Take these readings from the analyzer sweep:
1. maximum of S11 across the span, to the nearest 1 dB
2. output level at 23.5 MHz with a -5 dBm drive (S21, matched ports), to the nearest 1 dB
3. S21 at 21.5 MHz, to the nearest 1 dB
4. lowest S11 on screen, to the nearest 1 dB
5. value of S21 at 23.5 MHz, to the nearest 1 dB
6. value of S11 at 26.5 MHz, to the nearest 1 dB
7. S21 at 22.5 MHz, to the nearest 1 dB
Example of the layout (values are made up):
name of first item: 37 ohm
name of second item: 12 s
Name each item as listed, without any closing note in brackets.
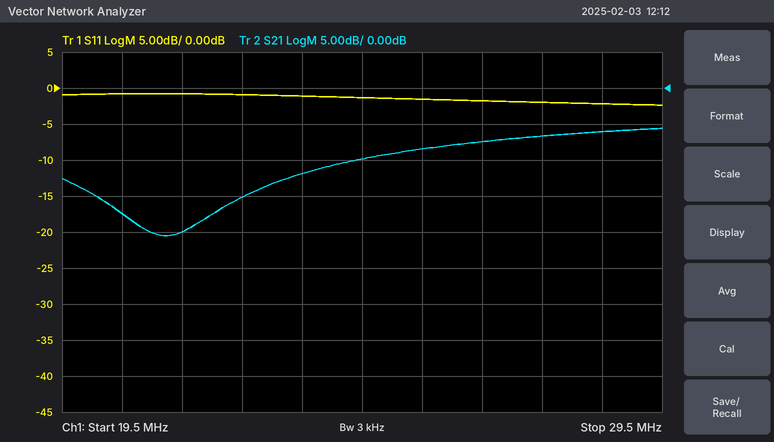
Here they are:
maximum of S11 across the span, to the nearest 1 dB: -1 dB
output level at 23.5 MHz with a -5 dBm drive (S21, matched ports), to the nearest 1 dB: -17 dBm
S21 at 21.5 MHz, to the nearest 1 dB: -20 dB
lowest S11 on screen, to the nearest 1 dB: -2 dB
value of S21 at 23.5 MHz, to the nearest 1 dB: -12 dB
value of S11 at 26.5 MHz, to the nearest 1 dB: -2 dB
S21 at 22.5 MHz, to the nearest 1 dB: -15 dB
